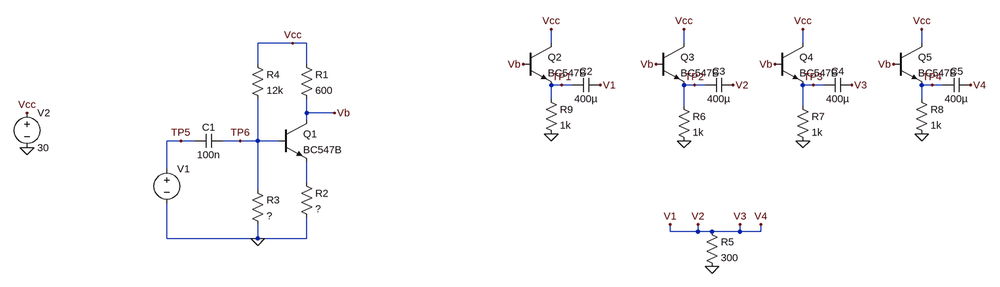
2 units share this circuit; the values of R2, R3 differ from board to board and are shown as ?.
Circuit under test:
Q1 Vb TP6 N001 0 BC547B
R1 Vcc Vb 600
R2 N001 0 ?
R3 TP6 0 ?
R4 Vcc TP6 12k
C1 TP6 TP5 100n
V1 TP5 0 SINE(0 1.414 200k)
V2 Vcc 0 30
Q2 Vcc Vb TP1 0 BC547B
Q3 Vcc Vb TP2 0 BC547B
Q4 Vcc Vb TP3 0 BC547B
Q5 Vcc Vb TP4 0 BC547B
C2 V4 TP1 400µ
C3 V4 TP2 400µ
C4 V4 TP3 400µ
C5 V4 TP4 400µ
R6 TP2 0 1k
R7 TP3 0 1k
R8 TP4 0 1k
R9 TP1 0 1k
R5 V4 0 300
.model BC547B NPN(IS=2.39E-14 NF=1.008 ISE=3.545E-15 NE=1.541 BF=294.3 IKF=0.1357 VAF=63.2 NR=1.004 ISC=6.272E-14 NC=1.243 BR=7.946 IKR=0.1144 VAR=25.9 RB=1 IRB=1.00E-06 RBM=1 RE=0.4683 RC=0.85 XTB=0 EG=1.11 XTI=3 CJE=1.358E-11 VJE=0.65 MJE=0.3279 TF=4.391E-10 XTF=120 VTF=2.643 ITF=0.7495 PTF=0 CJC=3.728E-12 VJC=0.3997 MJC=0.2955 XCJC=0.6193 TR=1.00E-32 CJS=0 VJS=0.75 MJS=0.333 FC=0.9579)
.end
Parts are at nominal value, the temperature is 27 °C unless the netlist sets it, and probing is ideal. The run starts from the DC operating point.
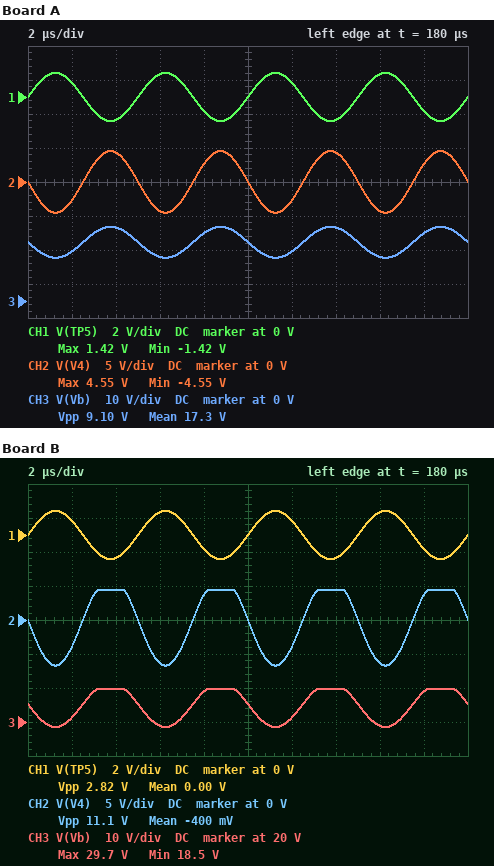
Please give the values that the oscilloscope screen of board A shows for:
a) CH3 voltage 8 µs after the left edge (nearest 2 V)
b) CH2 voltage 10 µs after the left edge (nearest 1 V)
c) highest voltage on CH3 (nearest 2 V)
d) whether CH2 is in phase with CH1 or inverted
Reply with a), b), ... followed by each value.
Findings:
a) 20 V
b) 0 V
c) 22 V
d) inverted
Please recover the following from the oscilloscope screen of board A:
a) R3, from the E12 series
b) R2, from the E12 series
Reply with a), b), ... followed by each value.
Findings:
a) 2.2 kΩ
b) 180 Ω
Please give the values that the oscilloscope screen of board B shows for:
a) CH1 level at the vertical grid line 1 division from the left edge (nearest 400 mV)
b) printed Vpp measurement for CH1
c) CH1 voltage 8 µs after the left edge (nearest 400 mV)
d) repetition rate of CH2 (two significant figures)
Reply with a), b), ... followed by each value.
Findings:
a) 800 mV
b) 2.82 V
c) -800 mV
d) 200 kHz
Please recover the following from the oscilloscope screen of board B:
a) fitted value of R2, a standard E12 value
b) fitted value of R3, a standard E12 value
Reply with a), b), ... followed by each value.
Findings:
a) 120 Ω
b) 680 Ω
